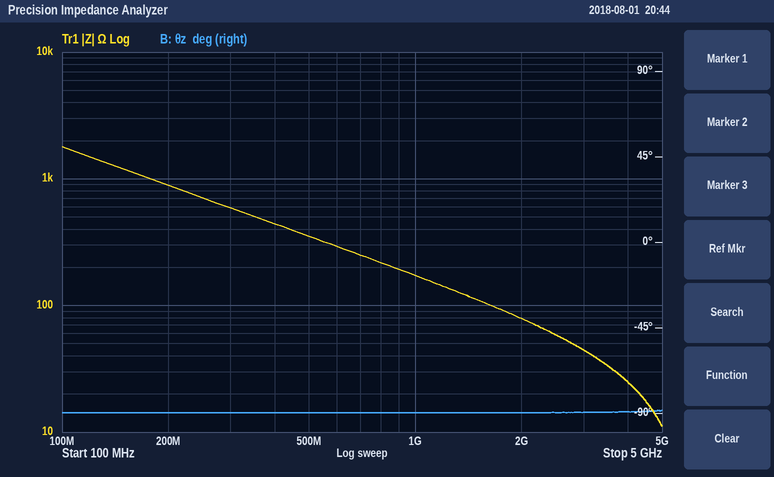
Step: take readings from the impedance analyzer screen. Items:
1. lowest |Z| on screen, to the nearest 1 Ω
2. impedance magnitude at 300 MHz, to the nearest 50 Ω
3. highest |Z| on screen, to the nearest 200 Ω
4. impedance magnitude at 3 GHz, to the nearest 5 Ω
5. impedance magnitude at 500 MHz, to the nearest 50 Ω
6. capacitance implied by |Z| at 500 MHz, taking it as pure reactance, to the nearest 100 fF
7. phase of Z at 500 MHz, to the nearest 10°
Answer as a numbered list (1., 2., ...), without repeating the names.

1. 11 Ω
2. 600 Ω
3. 1.8 kΩ
4. 45 Ω
5. 350 Ω
6. 900 fF
7. -90°
